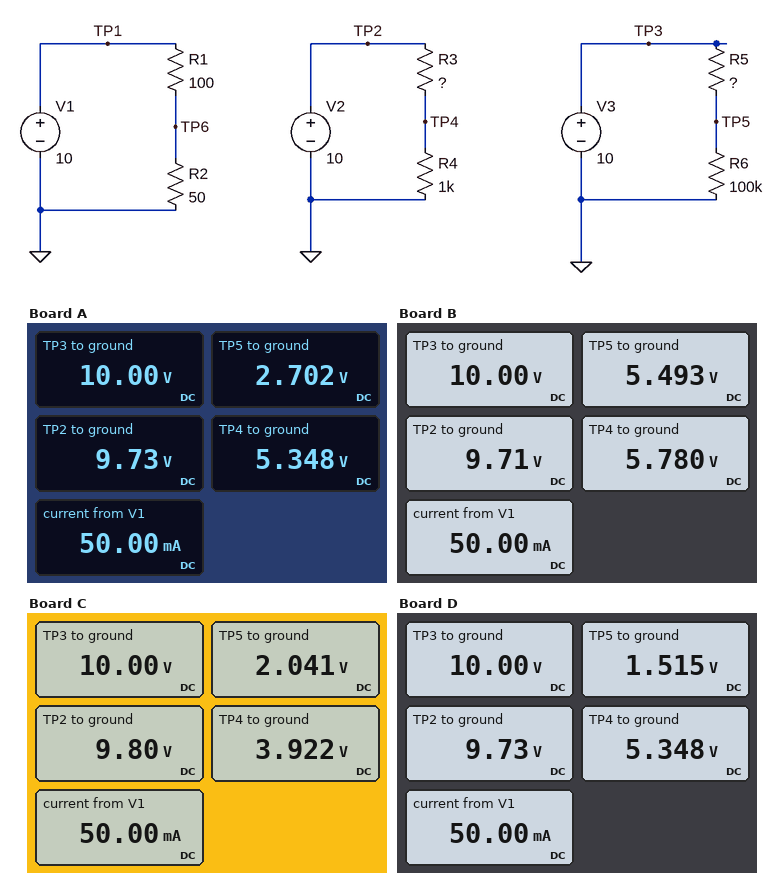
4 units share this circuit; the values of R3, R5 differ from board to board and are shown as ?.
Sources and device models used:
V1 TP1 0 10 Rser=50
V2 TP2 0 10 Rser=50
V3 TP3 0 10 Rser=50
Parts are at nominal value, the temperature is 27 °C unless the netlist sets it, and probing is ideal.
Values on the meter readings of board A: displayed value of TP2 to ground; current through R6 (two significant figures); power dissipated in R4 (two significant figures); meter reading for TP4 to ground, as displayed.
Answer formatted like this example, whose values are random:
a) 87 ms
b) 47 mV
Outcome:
a) 9.73 V
b) 27 µA
c) 29 mW
d) 5.348 V
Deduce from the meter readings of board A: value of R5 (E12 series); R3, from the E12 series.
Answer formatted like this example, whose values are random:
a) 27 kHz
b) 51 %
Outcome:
a) 270 kΩ
b) 820 Ω
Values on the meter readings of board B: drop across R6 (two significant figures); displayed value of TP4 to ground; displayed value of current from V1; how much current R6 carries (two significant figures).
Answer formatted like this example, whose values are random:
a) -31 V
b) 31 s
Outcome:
a) 5.5 V
b) 5.780 V
c) 50.00 mA
d) 55 µA
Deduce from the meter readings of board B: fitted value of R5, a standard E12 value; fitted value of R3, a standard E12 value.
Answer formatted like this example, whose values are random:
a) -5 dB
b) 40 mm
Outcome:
a) 82 kΩ
b) 680 Ω
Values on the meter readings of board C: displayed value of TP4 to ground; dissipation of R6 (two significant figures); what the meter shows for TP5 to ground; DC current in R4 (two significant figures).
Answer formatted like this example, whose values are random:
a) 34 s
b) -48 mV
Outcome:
a) 3.922 V
b) 42 µW
c) 2.041 V
d) 3.9 mA
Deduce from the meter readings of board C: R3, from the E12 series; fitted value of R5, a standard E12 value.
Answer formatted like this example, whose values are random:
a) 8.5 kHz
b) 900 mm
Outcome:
a) 1.5 kΩ
b) 390 kΩ
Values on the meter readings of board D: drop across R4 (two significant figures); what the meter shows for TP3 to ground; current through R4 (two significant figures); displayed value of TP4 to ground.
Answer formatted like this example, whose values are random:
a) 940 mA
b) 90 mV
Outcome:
a) 5.3 V
b) 10.00 V
c) 5.3 mA
d) 5.348 V
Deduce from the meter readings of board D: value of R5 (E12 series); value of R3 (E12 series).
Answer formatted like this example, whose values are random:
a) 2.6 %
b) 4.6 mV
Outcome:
a) 560 kΩ
b) 820 Ω
